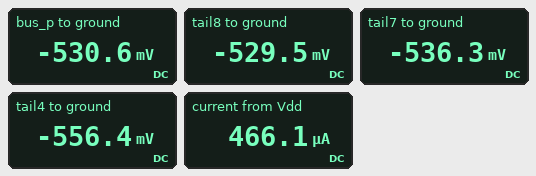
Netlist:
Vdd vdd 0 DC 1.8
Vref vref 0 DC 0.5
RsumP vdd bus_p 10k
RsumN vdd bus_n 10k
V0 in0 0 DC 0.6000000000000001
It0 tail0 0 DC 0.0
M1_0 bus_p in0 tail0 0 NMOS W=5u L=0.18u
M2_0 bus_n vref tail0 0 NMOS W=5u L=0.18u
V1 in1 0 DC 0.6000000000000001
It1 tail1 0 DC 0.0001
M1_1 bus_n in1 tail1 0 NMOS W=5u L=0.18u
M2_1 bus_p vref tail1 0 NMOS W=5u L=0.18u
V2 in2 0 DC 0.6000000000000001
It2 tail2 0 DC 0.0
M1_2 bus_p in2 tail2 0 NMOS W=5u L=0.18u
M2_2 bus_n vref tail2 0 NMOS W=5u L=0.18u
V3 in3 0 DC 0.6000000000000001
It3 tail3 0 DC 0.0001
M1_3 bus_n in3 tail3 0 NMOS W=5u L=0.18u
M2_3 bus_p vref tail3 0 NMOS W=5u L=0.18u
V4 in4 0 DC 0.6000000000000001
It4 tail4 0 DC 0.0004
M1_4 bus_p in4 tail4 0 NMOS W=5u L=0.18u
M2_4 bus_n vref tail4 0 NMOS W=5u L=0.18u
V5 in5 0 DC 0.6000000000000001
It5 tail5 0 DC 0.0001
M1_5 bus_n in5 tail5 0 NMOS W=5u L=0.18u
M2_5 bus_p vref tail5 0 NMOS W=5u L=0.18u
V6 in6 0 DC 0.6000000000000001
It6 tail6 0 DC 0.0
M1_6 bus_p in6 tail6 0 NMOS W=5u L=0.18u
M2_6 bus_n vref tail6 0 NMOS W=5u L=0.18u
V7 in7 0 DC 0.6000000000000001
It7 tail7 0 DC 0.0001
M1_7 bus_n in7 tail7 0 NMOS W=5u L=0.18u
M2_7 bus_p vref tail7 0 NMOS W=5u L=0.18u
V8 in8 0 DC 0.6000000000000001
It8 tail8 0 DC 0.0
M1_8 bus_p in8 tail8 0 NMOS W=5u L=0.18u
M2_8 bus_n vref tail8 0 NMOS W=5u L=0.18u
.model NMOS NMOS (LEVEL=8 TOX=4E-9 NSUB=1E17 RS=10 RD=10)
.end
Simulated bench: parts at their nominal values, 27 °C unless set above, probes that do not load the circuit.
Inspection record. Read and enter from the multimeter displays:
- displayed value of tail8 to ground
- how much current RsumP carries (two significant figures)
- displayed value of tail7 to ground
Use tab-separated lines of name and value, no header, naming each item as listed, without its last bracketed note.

displayed value of tail8 to ground	-529.5 mV
how much current RsumP carries	230 µA
displayed value of tail7 to ground	-536.3 mV
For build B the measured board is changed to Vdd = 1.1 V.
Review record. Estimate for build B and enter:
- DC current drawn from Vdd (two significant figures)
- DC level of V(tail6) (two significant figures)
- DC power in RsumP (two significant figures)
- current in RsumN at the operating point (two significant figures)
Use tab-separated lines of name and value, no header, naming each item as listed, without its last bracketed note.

DC current drawn from Vdd	330 µA
DC level of V(tail6)	-540 mV
DC power in RsumP	270 µW
current in RsumN at the operating point	160 µA
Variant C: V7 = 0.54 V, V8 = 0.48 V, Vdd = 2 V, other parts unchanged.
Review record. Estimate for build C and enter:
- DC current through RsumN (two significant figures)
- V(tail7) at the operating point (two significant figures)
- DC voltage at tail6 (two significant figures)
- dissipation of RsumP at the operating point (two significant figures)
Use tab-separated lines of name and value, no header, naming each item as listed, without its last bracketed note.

DC current through RsumN	250 µA
V(tail7) at the operating point	-530 mV
DC voltage at tail6	-530 mV
dissipation of RsumP at the operating point	640 µW
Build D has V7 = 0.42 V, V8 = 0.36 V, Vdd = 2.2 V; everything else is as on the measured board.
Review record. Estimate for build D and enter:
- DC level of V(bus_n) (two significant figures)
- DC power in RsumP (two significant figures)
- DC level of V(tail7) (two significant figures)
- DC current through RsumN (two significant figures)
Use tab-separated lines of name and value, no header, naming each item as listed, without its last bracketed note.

DC level of V(bus_n)	-520 mV
DC power in RsumP	740 µW
DC level of V(tail7)	-530 mV
DC current through RsumN	270 µA
